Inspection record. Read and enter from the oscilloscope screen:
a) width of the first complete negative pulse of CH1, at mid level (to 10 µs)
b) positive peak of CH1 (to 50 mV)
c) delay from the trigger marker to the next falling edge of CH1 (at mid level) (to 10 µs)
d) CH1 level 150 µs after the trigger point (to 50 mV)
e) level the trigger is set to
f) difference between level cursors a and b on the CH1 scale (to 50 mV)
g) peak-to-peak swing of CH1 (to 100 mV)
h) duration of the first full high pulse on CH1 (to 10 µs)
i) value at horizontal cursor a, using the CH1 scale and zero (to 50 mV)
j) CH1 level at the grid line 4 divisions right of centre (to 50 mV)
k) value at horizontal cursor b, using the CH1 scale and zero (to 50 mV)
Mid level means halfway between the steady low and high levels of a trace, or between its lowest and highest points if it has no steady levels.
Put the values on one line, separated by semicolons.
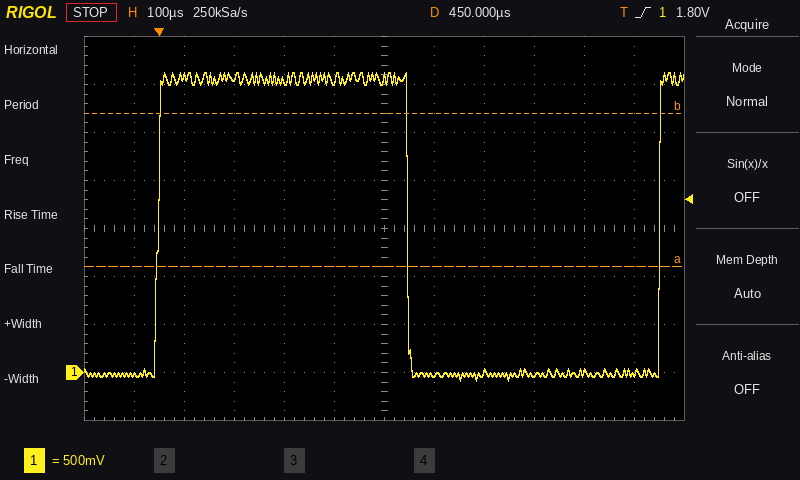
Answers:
500 µs; 3.10 V; 500 µs; 3.10 V; 1.80 V; 1.60 V; 3.20 V; 500 µs; 1.10 V; 0 mV; 2.70 V
